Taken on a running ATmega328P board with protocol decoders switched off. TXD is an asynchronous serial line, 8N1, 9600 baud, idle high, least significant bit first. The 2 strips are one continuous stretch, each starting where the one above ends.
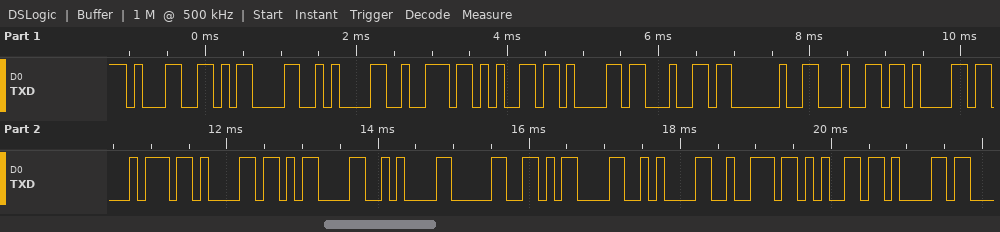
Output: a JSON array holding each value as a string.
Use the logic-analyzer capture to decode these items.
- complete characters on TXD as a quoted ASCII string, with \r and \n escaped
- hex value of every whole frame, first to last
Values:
["\"1\\r\\nread data\\r\\n0\\r\\nrea\"", "31 0D 0A 72 65 61 64 20 64 61 74 61 0D 0A 30 0D 0A 72 65 61"]
